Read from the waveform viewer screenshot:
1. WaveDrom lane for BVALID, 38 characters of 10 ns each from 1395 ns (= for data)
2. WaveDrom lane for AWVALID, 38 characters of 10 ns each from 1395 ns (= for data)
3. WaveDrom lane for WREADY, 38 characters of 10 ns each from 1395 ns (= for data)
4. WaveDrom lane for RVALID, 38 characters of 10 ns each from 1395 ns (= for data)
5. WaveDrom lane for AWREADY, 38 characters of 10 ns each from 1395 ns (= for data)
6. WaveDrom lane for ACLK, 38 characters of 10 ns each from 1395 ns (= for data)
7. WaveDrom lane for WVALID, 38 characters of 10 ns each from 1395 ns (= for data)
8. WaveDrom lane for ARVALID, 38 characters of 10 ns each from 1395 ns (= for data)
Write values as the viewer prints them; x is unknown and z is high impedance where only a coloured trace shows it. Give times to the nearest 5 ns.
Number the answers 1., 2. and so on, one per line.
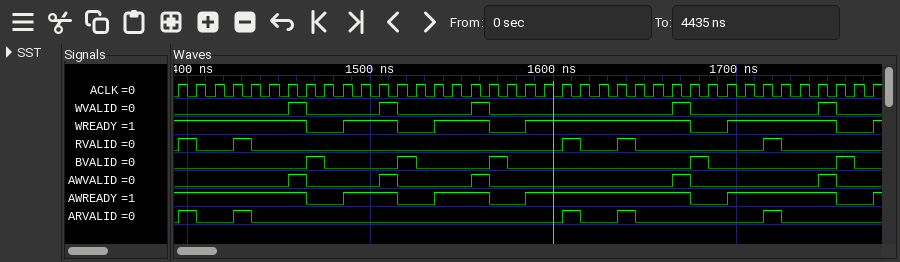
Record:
1. {name: 'BVALID', wave: '0......10...10...10.........10......10'}
2. {name: 'AWVALID', wave: '0.....10...10...10.........10......10.'}
3. {name: 'WREADY', wave: '1......0.1..0.1..0.1........0.1.....0.'}
4. {name: 'RVALID', wave: '10.10................10.10......10....'}
5. {name: 'AWREADY', wave: '1......0.1..0.1..0.1........0.1.....0.'}
6. {name: 'ACLK', wave: 'p.....................................'}
7. {name: 'WVALID', wave: '0.....10...10...10.........10......10.'}
8. {name: 'ARVALID', wave: '10.10................10.10......10....'}
